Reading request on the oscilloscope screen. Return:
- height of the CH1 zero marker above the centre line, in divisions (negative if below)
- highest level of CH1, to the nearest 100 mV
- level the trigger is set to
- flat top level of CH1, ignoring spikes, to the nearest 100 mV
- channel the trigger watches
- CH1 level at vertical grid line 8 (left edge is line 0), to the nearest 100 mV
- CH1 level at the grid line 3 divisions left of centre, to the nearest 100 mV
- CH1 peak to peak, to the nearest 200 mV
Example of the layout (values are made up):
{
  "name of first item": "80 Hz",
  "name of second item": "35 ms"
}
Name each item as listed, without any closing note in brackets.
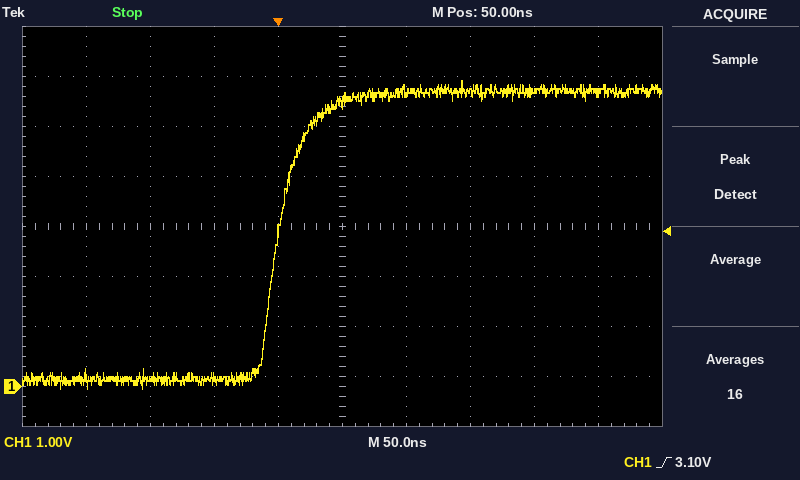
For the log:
{
  "height of the CH1 zero marker above the centre line, in divisions": "-3.2 div",
  "highest level of CH1, to the nearest 100 mV": "6.1 V",
  "level the trigger is set to": "3.10 V",
  "flat top level of CH1, ignoring spikes, to the nearest 100 mV": "5.9 V",
  "channel the trigger watches": "CH1",
  "CH1 level at vertical grid line 8 (left edge is line 0), to the nearest 100 mV": "5.9 V",
  "CH1 level at the grid line 3 divisions left of centre, to the nearest 100 mV": "200 mV",
  "CH1 peak to peak, to the nearest 200 mV": "6.2 V"
}
